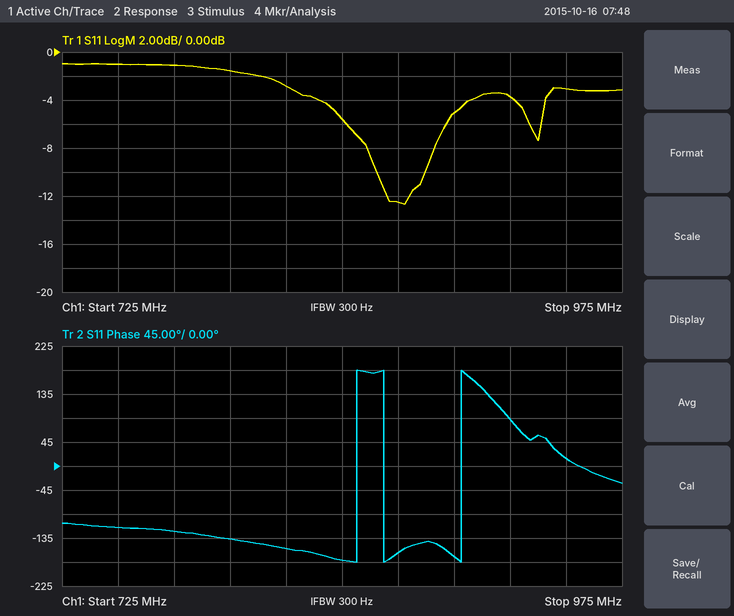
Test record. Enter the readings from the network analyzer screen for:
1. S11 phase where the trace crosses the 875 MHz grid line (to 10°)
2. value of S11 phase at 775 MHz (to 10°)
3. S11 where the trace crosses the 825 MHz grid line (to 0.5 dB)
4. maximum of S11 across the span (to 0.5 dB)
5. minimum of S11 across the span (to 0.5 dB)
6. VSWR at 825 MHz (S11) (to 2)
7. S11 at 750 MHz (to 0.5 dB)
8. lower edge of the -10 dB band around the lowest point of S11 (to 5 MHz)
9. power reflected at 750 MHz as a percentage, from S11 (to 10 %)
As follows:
-160°
-120°
-3.0 dB
-1.0 dB
-12.5 dB
6
-1.0 dB
865 MHz
80 %
